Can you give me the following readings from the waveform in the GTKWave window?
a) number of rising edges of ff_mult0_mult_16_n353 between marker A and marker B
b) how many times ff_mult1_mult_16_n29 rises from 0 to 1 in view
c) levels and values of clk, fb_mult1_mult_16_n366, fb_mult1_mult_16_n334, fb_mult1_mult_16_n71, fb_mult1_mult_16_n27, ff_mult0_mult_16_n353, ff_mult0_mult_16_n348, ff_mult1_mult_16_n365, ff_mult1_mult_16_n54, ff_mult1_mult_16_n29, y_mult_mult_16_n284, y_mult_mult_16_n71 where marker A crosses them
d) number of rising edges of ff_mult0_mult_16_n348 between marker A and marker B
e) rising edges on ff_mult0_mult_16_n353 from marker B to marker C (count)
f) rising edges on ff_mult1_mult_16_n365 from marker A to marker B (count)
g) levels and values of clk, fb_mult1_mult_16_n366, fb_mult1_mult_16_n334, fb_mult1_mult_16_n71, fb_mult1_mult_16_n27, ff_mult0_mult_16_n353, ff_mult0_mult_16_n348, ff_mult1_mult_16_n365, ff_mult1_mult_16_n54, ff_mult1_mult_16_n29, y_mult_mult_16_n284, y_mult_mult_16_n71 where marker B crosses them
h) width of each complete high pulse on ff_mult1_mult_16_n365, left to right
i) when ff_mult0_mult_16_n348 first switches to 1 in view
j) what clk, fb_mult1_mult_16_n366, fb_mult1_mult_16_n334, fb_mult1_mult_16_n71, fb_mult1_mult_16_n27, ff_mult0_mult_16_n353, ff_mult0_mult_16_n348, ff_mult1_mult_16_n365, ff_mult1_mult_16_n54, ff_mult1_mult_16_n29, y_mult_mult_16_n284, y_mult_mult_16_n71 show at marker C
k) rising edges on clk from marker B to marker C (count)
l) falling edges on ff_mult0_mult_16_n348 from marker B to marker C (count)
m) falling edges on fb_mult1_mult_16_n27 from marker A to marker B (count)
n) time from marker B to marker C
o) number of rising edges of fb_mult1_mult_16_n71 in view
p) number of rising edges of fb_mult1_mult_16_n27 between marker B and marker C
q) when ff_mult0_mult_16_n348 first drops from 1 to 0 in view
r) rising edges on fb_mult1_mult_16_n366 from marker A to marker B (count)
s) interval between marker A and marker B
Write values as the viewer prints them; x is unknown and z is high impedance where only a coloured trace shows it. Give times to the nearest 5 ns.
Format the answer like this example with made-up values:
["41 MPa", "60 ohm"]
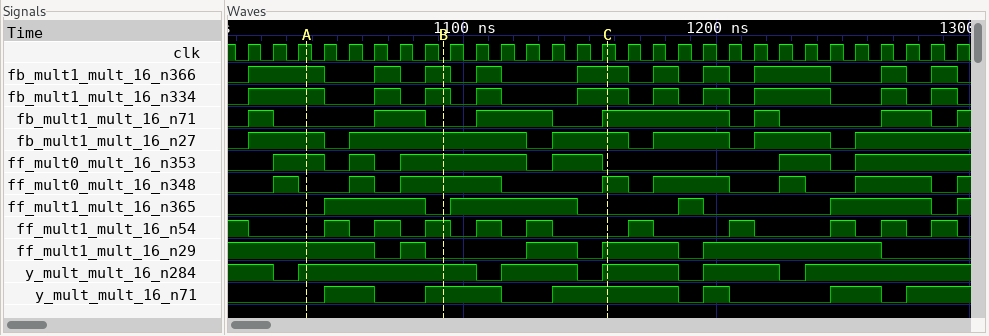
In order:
["2", "4", "clk=1, fb_mult1_mult_16_n366=1, fb_mult1_mult_16_n334=1, fb_mult1_mult_16_n71=0, fb_mult1_mult_16_n27=1, ff_mult0_mult_16_n353=1, ff_mult0_mult_16_n348=0, ff_mult1_mult_16_n365=0, ff_mult1_mult_16_n54=0, ff_mult1_mult_16_n29=1, y_mult_mult_16_n284=1, y_mult_mult_16_n71=0", "2", "1", "1", "clk=0, fb_mult1_mult_16_n366=1, fb_mult1_mult_16_n334=1, fb_mult1_mult_16_n71=0, fb_mult1_mult_16_n27=1, ff_mult0_mult_16_n353=1, ff_mult0_mult_16_n348=1, ff_mult1_mult_16_n365=0, ff_mult1_mult_16_n54=1, ff_mult1_mult_16_n29=0, y_mult_mult_16_n284=1, y_mult_mult_16_n71=1", "40 ns, 50 ns, 10 ns, 40 ns", "1025 ns", "clk=1, fb_mult1_mult_16_n366=1, fb_mult1_mult_16_n334=1, fb_mult1_mult_16_n71=1, fb_mult1_mult_16_n27=1, ff_mult0_mult_16_n353=0, ff_mult0_mult_16_n348=1, ff_mult1_mult_16_n365=0, ff_mult1_mult_16_n54=0, ff_mult1_mult_16_n29=1, y_mult_mult_16_n284=1, y_mult_mult_16_n71=1", "7", "1", "1", "65 ns", "7", "1", "1035 ns", "2", "55 ns"]
